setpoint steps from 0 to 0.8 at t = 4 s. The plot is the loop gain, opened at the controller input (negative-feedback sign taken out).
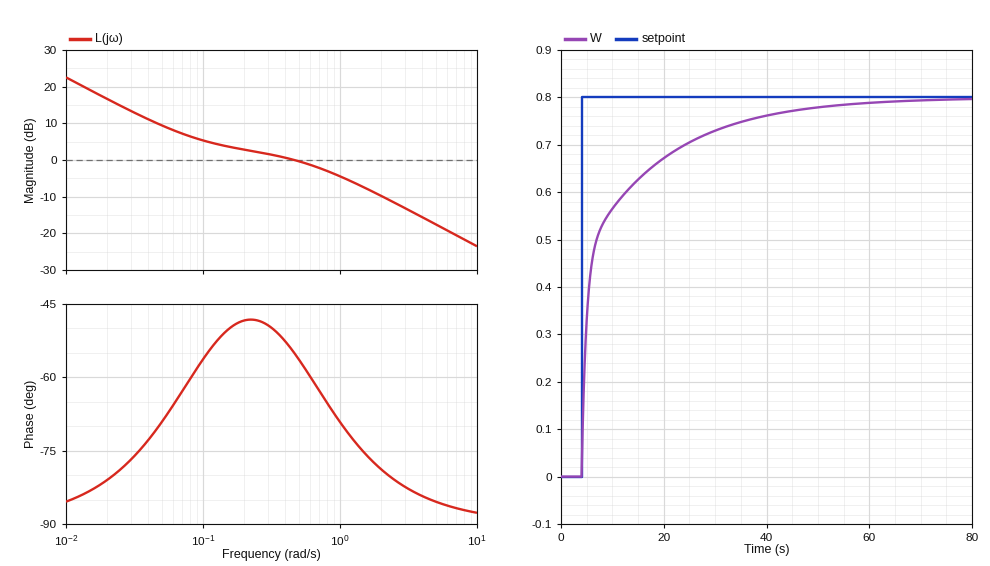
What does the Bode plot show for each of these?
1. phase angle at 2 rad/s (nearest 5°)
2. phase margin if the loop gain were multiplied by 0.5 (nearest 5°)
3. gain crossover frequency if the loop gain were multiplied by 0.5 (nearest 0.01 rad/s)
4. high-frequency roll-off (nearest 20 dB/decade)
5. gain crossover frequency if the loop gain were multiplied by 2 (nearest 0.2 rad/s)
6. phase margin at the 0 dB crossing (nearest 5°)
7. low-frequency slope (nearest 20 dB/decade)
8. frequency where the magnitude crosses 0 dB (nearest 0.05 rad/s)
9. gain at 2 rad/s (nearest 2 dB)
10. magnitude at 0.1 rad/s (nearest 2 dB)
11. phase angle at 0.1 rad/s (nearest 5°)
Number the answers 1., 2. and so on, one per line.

1. -80°
2. 120°
3. 0.09 rad/s
4. -20 dB/decade
5. 1.2 rad/s
6. 125°
7. -20 dB/decade
8. 0.45 rad/s
9. -10 dB
10. 6 dB
11. -55°
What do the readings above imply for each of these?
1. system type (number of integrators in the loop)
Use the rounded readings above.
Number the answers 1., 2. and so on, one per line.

1. 1
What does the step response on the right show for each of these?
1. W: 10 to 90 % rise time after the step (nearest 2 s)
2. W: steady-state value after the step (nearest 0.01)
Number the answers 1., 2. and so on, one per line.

1. 24 s
2. 0.80
